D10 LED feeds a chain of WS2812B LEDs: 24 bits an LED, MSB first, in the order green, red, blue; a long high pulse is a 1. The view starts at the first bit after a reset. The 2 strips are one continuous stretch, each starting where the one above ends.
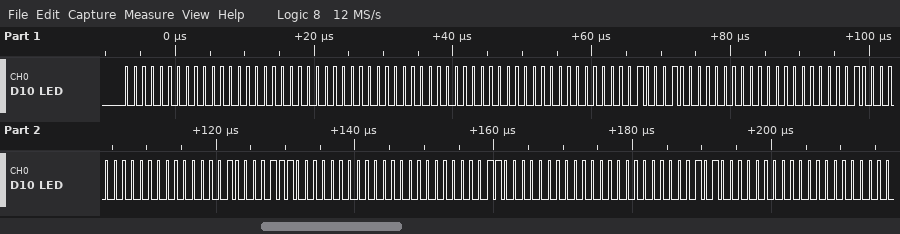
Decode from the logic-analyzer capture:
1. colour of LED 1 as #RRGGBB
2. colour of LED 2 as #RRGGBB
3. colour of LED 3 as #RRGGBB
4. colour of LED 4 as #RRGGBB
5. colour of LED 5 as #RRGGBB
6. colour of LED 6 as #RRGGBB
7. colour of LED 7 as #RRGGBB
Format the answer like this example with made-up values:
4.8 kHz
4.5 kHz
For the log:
#000000
#000000
#110000
#080000
#0E0100
#060000
#050000
